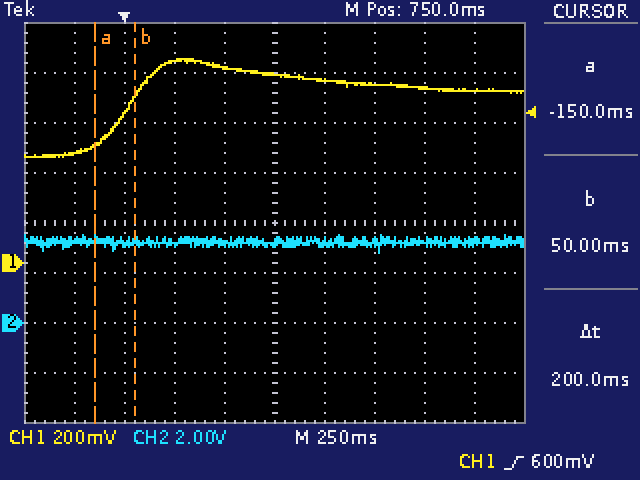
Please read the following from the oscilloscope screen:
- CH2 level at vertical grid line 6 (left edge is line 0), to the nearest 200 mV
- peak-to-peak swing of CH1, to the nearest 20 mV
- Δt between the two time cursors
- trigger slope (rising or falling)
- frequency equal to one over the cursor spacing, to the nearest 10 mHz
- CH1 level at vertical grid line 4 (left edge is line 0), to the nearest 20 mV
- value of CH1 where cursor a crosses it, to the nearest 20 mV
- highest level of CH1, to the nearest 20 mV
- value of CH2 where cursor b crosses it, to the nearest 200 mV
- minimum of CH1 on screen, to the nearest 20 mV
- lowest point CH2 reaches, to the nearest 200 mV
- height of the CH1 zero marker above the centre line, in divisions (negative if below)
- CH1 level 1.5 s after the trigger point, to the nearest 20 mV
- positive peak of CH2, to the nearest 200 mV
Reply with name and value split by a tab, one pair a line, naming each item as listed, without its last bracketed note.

CH2 level at vertical grid line 6 (left edge is line 0), to the nearest 200 mV	3.2 V
peak-to-peak swing of CH1, to the nearest 20 mV	400 mV
Δt between the two time cursors	200 ms
trigger slope	rising
frequency equal to one over the cursor spacing, to the nearest 10 mHz	5.00 Hz
CH1 level at vertical grid line 4 (left edge is line 0), to the nearest 20 mV	780 mV
value of CH1 where cursor a crosses it, to the nearest 20 mV	480 mV
highest level of CH1, to the nearest 20 mV	820 mV
value of CH2 where cursor b crosses it, to the nearest 200 mV	3.2 V
minimum of CH1 on screen, to the nearest 20 mV	420 mV
lowest point CH2 reaches, to the nearest 200 mV	2.8 V
height of the CH1 zero marker above the centre line, in divisions	-0.8 div
CH1 level 1.5 s after the trigger point, to the nearest 20 mV	700 mV
positive peak of CH2, to the nearest 200 mV	3.6 V
